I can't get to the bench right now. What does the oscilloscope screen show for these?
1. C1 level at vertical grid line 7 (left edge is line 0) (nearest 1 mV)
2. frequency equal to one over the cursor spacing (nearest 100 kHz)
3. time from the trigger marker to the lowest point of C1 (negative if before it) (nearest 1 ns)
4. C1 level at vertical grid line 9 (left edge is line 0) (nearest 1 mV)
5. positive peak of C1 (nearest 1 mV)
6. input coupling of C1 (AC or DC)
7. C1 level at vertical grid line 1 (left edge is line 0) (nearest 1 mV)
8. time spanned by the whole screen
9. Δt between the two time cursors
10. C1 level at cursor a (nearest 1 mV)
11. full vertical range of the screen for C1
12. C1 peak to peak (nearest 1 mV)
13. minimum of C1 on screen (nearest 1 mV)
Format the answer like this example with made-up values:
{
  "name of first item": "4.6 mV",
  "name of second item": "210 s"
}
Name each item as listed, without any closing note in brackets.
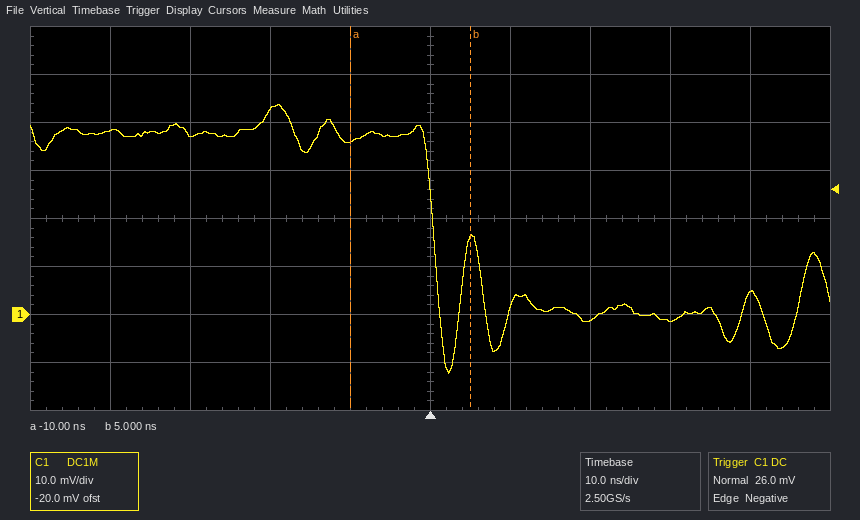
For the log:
{
  "C1 level at vertical grid line 7 (left edge is line 0)": "-1 mV",
  "frequency equal to one over the cursor spacing": "66.7 MHz",
  "time from the trigger marker to the lowest point of C1 (negative if before it)": "+2 ns",
  "C1 level at vertical grid line 9 (left edge is line 0)": "4 mV",
  "positive peak of C1": "44 mV",
  "input coupling of C1": "DC",
  "C1 level at vertical grid line 1 (left edge is line 0)": "38 mV",
  "time spanned by the whole screen": "100 ns",
  "Δt between the two time cursors": "15 ns",
  "C1 level at cursor a": "36 mV",
  "full vertical range of the screen for C1": "80 mV",
  "C1 peak to peak": "56 mV",
  "minimum of C1 on screen": "-12 mV"
}
